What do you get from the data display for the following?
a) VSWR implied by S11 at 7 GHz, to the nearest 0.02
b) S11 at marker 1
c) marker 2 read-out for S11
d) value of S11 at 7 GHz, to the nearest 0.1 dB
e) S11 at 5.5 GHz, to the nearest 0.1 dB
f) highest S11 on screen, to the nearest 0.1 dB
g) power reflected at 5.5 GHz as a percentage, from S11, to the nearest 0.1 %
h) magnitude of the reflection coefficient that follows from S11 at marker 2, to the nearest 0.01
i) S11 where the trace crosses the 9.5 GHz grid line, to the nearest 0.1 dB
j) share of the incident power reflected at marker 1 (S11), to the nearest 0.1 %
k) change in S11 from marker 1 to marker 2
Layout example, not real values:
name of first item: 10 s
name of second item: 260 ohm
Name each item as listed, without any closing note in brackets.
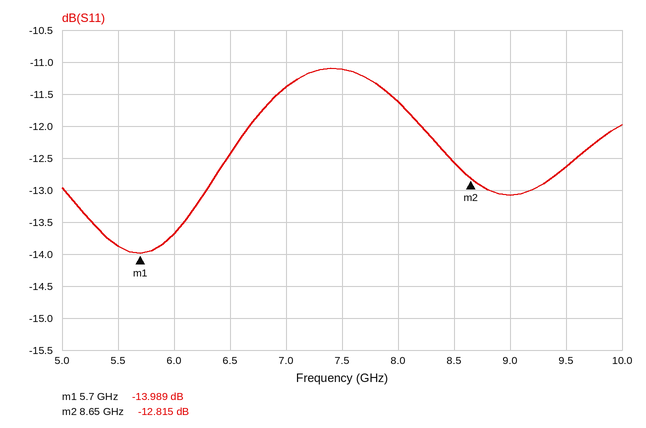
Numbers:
VSWR implied by S11 at 7 GHz, to the nearest 0.02: 1.74
S11 at marker 1: -13.989 dB
marker 2 read-out for S11: -12.815 dB
value of S11 at 7 GHz, to the nearest 0.1 dB: -11.4 dB
S11 at 5.5 GHz, to the nearest 0.1 dB: -13.9 dB
highest S11 on screen, to the nearest 0.1 dB: -11.1 dB
power reflected at 5.5 GHz as a percentage, from S11, to the nearest 0.1 %: 4.1 %
magnitude of the reflection coefficient that follows from S11 at marker 2, to the nearest 0.01: 0.23
S11 where the trace crosses the 9.5 GHz grid line, to the nearest 0.1 dB: -12.6 dB
share of the incident power reflected at marker 1 (S11), to the nearest 0.1 %: 4.0 %
change in S11 from marker 1 to marker 2: 1.174 dB
